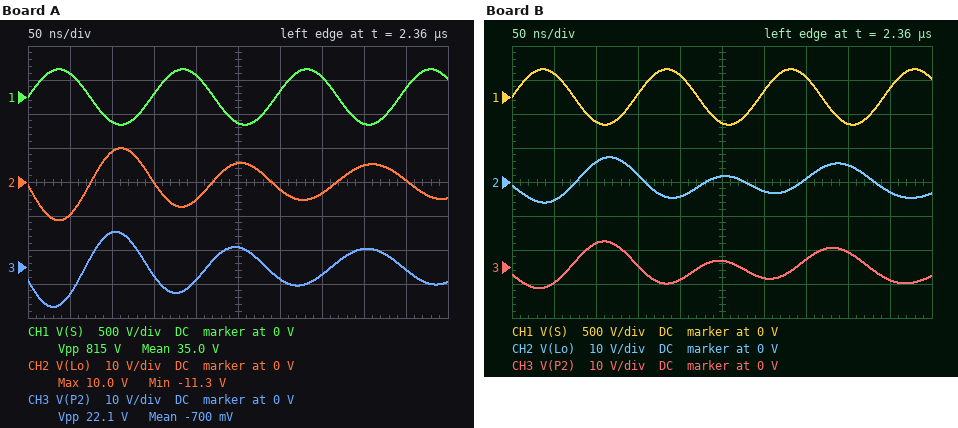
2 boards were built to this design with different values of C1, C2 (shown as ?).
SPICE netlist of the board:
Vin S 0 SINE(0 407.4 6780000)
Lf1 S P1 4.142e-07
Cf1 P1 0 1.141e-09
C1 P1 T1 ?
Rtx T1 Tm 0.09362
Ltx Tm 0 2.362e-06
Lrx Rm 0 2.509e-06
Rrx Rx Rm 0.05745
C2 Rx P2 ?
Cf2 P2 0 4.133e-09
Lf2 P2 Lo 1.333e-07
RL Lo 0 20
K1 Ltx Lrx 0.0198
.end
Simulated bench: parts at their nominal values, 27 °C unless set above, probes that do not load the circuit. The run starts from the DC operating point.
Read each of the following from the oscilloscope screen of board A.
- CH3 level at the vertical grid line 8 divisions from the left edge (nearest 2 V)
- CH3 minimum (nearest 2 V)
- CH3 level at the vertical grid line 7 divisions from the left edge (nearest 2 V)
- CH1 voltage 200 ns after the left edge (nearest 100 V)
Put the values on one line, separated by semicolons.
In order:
6 V; -12 V; -2 V; 300 V
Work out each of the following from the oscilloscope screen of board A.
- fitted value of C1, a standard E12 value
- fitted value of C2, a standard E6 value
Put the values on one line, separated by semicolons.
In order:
470 pF; 330 pF
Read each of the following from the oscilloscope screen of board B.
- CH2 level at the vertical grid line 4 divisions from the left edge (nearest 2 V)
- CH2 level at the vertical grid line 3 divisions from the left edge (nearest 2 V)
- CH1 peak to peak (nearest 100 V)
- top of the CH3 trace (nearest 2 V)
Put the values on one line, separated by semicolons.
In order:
-4 V; 2 V; 800 V; 8 V
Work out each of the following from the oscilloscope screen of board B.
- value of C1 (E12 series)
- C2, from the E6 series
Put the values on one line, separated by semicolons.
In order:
560 pF; 470 pF
